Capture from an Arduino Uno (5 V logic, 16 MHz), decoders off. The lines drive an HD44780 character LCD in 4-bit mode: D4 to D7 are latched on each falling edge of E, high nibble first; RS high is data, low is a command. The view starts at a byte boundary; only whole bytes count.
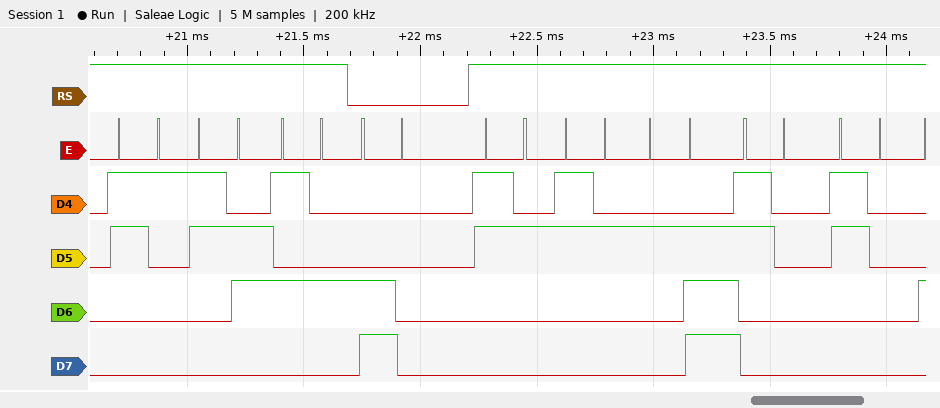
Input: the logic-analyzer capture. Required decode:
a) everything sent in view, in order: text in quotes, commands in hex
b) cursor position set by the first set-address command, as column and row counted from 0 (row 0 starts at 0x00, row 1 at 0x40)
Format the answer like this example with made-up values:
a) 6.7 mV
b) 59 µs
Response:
a) "16T" 0xC0 "22.00"
b) column 0, row 1
